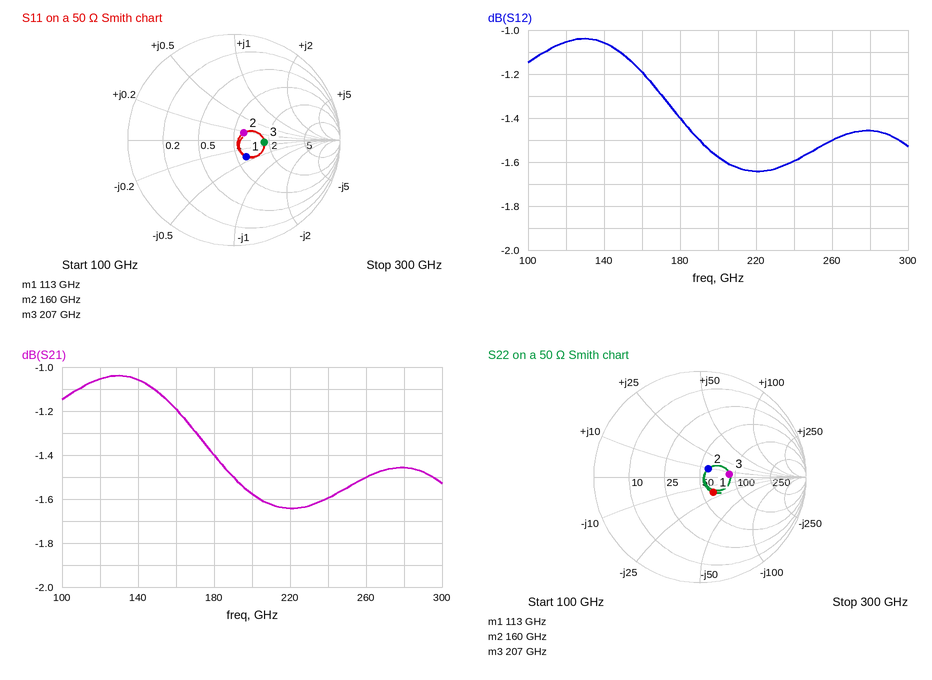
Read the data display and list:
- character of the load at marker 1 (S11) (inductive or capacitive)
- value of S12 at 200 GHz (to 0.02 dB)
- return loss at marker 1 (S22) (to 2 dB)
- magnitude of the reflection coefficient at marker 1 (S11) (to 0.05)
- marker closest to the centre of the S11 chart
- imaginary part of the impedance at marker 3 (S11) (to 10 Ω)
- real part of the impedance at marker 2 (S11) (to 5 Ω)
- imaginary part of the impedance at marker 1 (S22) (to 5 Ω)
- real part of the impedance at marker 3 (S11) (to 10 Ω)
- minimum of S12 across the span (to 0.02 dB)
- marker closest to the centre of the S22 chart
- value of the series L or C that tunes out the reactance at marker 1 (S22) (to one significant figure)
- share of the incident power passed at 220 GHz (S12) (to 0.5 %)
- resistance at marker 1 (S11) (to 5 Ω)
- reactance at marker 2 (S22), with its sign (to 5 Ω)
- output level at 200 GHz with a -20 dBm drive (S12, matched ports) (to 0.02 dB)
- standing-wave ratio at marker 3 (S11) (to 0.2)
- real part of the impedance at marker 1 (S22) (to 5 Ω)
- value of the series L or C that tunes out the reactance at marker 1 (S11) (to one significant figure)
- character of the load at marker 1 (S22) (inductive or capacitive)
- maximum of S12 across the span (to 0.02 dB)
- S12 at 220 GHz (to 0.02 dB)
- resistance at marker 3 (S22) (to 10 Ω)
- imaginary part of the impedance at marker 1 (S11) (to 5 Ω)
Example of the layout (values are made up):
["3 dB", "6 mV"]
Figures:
["capacitive", "-1.58 dB", "14 dB", "0.20", "marker 2", "0 Ω", "60 Ω", "-20 Ω", "90 Ω", "-1.64 dB", "marker 2", "30 pH", "68.5 %", "60 Ω", "+10 Ω", "-21.58 dBm", "1.8", "60 Ω", "30 pH", "capacitive", "-1.04 dB", "-1.64 dB", "90 Ω", "-20 Ω"]
